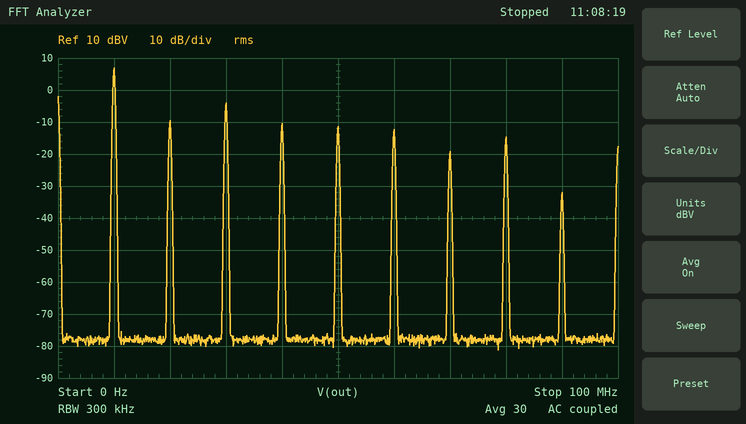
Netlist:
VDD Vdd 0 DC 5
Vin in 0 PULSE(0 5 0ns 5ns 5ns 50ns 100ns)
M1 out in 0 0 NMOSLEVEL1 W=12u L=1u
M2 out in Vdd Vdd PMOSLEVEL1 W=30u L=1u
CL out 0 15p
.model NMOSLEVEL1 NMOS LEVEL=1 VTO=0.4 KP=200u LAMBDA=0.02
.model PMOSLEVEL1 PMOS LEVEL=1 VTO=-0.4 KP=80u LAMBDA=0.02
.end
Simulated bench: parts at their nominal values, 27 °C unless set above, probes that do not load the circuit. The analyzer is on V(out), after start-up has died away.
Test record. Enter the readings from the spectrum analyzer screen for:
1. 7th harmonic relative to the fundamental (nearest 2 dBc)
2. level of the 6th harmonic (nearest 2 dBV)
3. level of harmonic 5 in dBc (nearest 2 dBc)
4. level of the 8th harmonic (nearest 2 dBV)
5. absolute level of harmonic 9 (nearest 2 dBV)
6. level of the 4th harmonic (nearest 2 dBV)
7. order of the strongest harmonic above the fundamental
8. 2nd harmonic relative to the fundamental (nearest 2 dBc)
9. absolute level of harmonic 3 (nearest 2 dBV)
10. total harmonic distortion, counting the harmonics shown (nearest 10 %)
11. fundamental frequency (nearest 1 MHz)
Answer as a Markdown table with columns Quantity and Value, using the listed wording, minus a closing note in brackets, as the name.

| Quantity | Value |
|---|---|
| 7th harmonic relative to the fundamental | -26 dBc |
| level of the 6th harmonic | -12 dBV |
| level of harmonic 5 in dBc | -18 dBc |
| level of the 8th harmonic | -14 dBV |
| absolute level of harmonic 9 | -32 dBV |
| level of the 4th harmonic | -10 dBV |
| order of the strongest harmonic above the fundamental | 3 |
| 2nd harmonic relative to the fundamental | -16 dBc |
| absolute level of harmonic 3 | -4 dBV |
| total harmonic distortion, counting the harmonics shown | 40 % |
| fundamental frequency | 10 MHz |
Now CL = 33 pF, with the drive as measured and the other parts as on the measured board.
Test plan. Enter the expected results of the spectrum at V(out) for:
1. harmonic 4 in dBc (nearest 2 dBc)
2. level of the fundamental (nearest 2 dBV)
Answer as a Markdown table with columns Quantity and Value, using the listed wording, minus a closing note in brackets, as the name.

| Quantity | Value |
|---|---|
| harmonic 4 in dBc | -20 dBc |
| level of the fundamental | 6 dBV |
